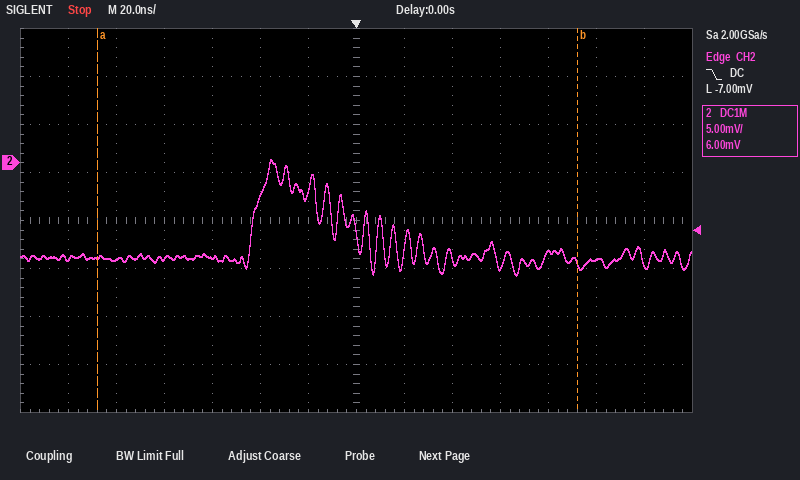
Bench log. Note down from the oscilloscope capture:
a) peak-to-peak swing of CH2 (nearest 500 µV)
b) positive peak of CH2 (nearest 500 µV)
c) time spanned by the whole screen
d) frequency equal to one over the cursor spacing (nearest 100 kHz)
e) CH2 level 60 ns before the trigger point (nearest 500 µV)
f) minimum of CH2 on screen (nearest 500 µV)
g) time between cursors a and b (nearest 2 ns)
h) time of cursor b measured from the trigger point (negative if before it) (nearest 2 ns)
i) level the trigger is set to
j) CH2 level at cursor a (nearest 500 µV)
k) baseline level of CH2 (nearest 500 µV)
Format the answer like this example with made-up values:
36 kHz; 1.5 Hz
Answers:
12.0 mV; 500 µV; 280 ns; 5.0 MHz; -10.0 mV; -11.5 mV; 200 ns; +92 ns; -7.00 mV; -10.0 mV; -10.0 mV
